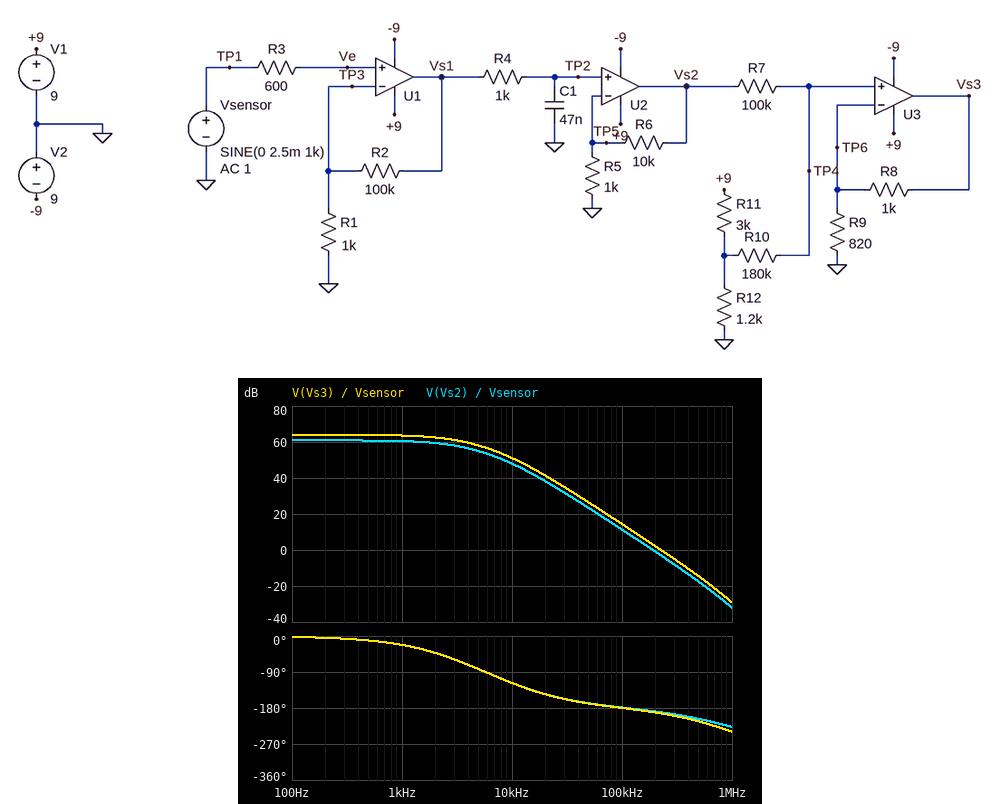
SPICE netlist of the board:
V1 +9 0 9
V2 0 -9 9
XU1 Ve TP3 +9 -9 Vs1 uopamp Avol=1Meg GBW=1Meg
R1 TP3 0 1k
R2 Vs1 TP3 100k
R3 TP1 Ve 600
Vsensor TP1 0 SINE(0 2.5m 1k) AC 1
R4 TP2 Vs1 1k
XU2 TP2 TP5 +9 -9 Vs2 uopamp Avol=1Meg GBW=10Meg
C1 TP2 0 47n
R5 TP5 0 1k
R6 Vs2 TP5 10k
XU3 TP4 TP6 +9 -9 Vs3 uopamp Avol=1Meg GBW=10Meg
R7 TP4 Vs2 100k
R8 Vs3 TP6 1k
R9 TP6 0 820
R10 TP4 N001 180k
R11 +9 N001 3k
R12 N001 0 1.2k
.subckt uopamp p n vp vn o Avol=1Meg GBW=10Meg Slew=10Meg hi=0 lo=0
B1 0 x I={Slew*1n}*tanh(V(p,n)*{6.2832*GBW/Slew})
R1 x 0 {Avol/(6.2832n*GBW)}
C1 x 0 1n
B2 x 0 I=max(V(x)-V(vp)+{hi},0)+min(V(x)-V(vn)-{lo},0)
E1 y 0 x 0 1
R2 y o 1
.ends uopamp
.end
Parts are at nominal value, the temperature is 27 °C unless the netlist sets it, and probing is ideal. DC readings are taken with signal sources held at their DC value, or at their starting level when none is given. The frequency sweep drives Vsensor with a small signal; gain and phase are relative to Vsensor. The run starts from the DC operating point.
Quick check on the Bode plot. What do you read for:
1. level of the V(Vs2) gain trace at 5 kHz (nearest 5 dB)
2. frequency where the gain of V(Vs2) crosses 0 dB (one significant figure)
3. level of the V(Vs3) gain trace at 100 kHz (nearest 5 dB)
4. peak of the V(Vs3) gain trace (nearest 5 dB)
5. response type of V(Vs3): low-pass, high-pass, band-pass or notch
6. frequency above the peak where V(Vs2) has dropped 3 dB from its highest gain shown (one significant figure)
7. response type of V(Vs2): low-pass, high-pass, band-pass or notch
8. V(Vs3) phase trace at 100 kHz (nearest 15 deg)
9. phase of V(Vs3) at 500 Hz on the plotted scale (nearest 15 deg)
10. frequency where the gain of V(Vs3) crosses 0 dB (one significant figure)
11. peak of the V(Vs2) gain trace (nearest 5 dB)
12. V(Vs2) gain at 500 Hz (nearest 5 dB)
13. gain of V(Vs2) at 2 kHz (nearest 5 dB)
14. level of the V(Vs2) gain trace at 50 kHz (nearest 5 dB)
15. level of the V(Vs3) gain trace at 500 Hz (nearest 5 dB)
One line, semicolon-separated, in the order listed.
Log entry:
55 dB; 200 kHz; 15 dB; 65 dB; low-pass; 3 kHz; low-pass; -180 deg; -15 deg; 200 kHz; 60 dB; 60 dB; 60 dB; 25 dB; 65 dB
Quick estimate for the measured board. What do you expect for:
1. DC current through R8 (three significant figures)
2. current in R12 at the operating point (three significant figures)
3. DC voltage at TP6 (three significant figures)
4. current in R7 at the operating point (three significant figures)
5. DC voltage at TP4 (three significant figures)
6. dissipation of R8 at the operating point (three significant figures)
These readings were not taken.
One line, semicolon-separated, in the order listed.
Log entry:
1.12 mA; 2.14 mA; 916 mV; 9.16 µA; 916 mV; 1.25 mW
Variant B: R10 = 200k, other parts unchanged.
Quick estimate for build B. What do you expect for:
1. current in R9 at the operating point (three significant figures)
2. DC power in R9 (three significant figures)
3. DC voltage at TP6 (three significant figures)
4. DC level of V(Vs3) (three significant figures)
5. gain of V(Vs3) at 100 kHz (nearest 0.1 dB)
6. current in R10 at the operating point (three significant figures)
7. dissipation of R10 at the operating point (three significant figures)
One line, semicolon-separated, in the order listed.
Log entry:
1.04 mA; 891 µW; 855 mV; 1.90 V; 14.7 dB; 8.55 µA; 14.6 µW
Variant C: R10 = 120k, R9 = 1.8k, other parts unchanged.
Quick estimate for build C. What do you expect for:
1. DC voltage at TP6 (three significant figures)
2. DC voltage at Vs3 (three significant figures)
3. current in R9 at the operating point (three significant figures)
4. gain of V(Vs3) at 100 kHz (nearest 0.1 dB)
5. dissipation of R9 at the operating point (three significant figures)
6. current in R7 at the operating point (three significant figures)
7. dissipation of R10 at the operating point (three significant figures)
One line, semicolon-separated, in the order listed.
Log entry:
1.16 V; 1.81 V; 647 µA; 9.9 dB; 753 µW; 11.6 µA; 16.3 µW
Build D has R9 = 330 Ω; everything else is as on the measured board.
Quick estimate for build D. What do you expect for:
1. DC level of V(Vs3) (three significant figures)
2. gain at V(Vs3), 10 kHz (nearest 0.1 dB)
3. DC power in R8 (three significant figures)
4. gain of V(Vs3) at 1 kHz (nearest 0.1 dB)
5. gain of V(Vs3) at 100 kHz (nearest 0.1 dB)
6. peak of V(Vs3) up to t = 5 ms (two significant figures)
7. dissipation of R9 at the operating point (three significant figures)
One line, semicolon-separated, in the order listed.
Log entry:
3.69 V; 56.3 dB; 7.70 mW; 68.8 dB; 19.6 dB; 9.0 V; 2.54 mW
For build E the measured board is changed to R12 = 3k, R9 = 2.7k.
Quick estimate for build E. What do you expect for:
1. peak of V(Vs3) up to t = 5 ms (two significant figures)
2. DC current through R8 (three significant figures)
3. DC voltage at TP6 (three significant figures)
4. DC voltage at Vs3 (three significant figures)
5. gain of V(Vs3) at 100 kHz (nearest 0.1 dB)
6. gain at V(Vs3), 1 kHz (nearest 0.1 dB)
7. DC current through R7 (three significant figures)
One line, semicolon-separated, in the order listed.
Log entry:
4.5 V; 592 µA; 1.60 V; 2.19 V; 10.2 dB; 59.4 dB; 16.0 µA
